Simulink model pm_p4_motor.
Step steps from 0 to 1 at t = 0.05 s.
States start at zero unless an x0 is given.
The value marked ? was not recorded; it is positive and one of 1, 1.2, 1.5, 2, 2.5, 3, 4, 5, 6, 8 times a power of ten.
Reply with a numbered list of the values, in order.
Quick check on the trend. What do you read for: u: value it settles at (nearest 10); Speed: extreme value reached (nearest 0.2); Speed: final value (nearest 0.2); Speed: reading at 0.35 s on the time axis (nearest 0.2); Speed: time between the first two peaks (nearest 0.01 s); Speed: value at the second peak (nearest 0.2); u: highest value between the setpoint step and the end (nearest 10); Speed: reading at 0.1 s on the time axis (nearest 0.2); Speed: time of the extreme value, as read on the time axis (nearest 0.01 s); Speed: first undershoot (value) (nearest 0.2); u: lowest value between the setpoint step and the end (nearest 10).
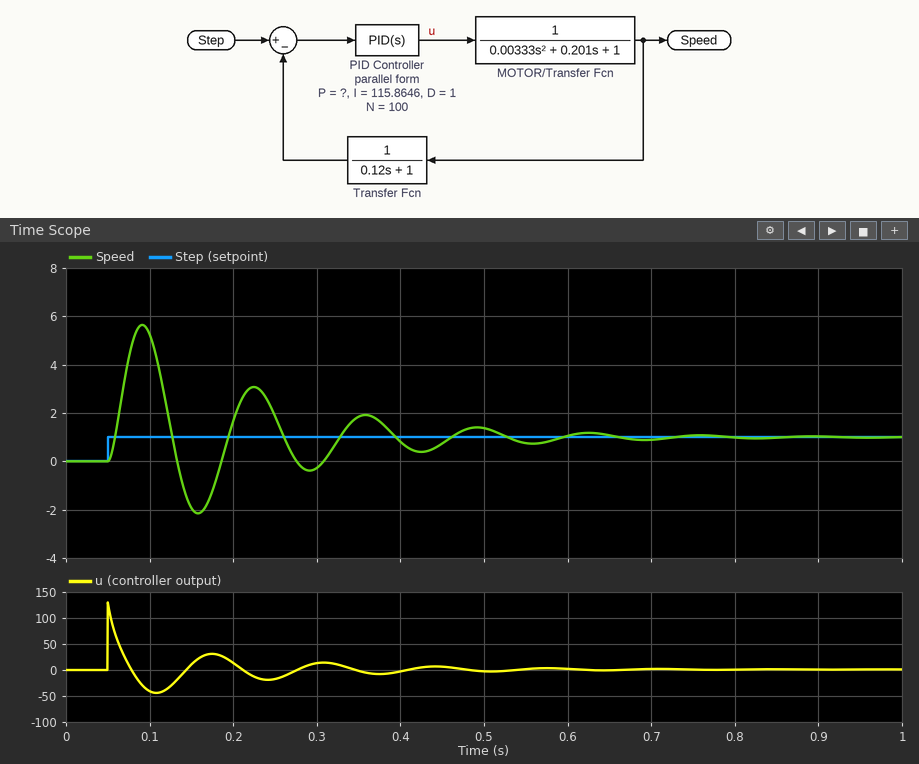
1. 0
2. 5.6
3. 1.0
4. 1.8
5. 0.13 s
6. 3.0
7. 130
8. 5.2
9. 0.09 s
10. -2.2
11. -40
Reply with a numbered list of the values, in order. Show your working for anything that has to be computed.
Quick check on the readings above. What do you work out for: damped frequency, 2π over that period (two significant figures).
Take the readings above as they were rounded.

1. 2π / 0.13 = 48 rad/s
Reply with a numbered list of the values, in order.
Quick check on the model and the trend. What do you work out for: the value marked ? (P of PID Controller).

1. 30
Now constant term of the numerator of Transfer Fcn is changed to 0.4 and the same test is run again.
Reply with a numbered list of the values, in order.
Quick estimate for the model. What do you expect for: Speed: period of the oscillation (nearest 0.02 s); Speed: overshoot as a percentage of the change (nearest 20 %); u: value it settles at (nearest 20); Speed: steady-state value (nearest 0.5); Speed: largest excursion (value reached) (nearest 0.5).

1. 0.24 s
2. 220 %
3. 0
4. 2.5
5. 8.0
